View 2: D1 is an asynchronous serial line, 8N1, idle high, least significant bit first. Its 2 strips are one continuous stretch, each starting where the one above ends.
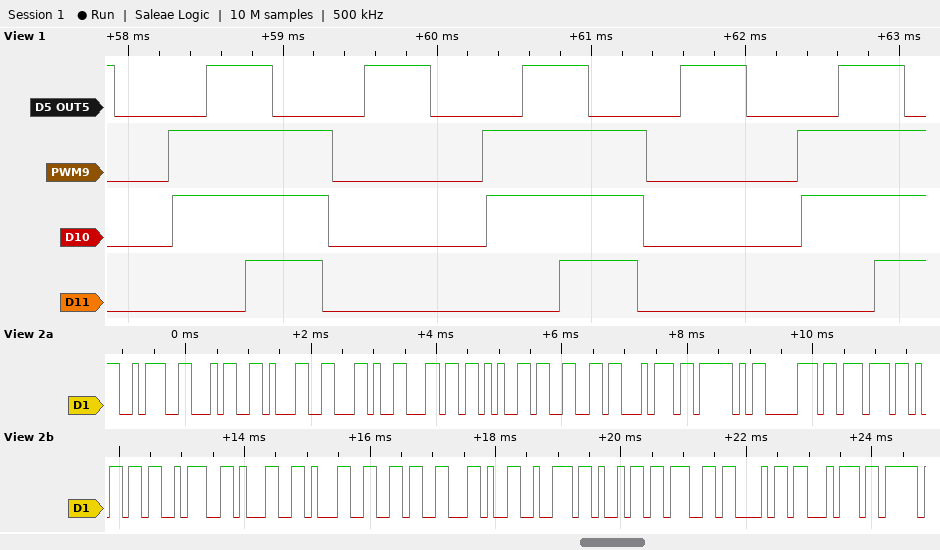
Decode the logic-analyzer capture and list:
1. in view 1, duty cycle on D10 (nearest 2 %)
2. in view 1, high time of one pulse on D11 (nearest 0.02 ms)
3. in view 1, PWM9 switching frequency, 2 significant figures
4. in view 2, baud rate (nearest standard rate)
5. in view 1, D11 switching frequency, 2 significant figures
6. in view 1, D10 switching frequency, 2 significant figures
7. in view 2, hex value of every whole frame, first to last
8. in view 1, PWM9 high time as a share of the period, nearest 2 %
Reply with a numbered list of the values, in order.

1. 50 %
2. 0.50 ms
3. 490 Hz
4. 9600 baud
5. 490 Hz
6. 490 Hz
7. 0x3A 0x34 0x31 0x2C 0x6C 0x65 0x66 0x74 0x5F 0x70 0x77 0x6D 0x3A 0x31 0x31 0x36 0x2C 0x72 0x69 0x67 0x68 0x74
8. 52 %
